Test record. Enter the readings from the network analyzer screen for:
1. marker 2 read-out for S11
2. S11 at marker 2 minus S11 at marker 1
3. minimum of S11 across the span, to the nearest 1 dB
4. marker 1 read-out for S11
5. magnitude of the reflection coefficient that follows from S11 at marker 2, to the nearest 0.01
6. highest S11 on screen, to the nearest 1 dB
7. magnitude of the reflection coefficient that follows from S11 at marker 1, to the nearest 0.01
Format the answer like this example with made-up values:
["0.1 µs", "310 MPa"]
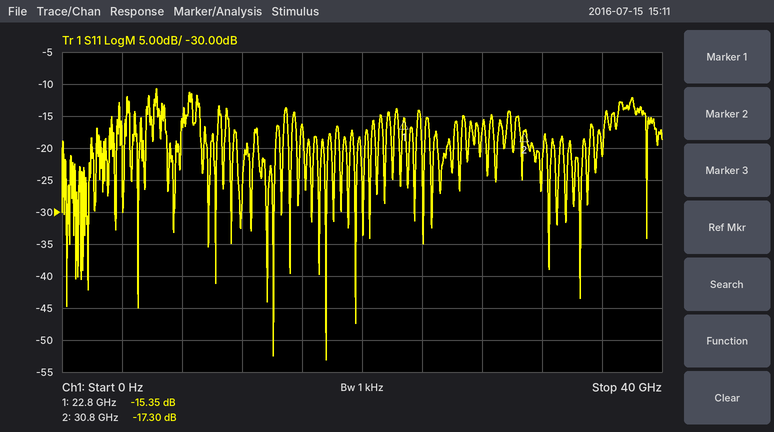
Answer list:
["-17.30 dB", "-1.95 dB", "-53 dB", "-15.35 dB", "0.14", "-11 dB", "0.17"]
